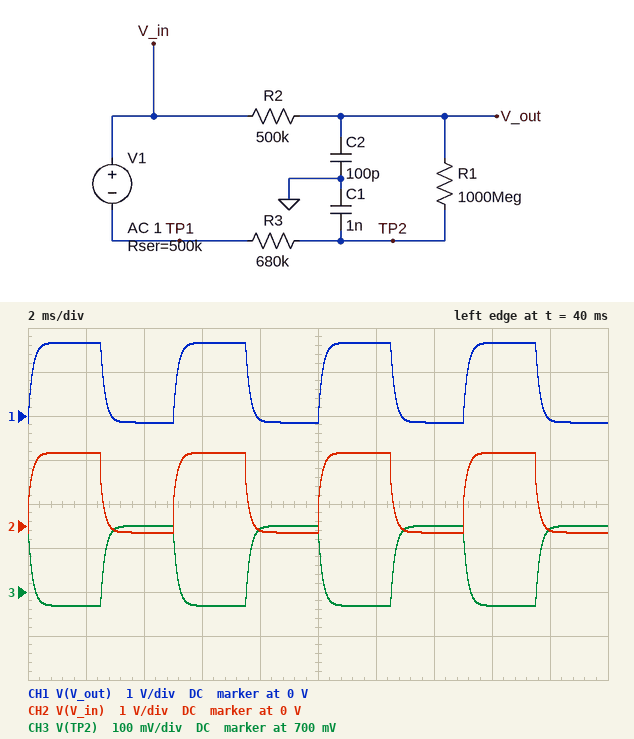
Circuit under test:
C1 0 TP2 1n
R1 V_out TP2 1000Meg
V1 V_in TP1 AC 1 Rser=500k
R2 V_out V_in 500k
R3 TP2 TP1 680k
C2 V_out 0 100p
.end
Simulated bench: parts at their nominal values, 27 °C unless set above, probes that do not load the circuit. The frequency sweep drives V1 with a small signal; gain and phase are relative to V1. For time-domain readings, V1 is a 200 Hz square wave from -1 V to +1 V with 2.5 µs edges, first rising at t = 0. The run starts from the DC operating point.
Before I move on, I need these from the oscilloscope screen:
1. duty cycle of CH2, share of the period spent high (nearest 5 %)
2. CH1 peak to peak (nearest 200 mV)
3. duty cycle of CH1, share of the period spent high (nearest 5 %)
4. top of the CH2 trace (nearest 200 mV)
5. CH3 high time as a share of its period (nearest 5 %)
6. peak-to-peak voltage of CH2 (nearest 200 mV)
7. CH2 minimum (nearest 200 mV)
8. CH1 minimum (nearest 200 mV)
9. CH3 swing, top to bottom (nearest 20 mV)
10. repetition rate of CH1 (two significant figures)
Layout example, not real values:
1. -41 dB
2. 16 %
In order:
1. 50 %
2. 1.8 V
3. 50 %
4. 1.6 V
5. 50 %
6. 1.8 V
7. -200 mV
8. -200 mV
9. 180 mV
10. 200 Hz
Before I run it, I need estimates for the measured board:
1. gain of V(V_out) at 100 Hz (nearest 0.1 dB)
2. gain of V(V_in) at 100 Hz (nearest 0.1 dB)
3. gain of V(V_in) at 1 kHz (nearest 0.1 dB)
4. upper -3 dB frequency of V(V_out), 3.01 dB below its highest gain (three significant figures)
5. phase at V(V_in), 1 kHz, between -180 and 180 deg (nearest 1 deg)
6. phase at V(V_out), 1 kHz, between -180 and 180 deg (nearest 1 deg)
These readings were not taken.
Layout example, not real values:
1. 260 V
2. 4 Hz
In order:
1. -0.9 dB
2. -0.9 dB
3. -3.3 dB
4. 1.04 kHz
5. -26 deg
6. -44 deg
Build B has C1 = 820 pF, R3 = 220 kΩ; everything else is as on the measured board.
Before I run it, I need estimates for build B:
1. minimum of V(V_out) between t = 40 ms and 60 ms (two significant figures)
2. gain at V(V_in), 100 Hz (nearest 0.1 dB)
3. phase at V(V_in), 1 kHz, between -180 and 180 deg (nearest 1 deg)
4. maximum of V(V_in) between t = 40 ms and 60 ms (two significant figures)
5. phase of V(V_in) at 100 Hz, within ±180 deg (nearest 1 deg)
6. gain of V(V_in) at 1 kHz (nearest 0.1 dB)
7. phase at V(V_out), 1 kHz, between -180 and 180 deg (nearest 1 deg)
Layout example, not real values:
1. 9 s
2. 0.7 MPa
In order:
1. 160 mV
2. -1.0 dB
3. -17 deg
4. 1.9 V
5. -2 deg
6. -2.3 dB
7. -34 deg
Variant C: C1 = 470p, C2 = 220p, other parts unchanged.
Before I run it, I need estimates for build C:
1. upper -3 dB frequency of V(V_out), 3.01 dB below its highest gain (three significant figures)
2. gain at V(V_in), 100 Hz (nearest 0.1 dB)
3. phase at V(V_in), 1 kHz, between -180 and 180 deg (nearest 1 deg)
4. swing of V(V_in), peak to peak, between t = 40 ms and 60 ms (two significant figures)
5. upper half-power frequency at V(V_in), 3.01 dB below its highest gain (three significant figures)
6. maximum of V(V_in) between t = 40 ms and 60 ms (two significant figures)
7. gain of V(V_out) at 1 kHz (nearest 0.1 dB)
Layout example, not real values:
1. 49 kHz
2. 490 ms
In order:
1. 633 Hz
2. -3.4 dB
3. -23 deg
4. 1.4 V
5. 806 Hz
6. 1.2 V
7. -8.8 dB
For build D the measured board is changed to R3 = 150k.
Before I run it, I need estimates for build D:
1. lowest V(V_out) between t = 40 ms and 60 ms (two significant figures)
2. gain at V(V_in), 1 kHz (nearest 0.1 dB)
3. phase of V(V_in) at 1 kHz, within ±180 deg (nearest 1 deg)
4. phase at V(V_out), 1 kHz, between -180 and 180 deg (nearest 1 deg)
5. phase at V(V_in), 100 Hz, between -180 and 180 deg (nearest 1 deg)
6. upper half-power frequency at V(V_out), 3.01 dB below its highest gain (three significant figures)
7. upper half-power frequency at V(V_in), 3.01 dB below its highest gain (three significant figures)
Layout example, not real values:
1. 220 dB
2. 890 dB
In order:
1. 740 mV
2. -2.0 dB
3. -16 deg
4. -33 deg
5. -2 deg
6. 1.52 kHz
7. 2.07 kHz
